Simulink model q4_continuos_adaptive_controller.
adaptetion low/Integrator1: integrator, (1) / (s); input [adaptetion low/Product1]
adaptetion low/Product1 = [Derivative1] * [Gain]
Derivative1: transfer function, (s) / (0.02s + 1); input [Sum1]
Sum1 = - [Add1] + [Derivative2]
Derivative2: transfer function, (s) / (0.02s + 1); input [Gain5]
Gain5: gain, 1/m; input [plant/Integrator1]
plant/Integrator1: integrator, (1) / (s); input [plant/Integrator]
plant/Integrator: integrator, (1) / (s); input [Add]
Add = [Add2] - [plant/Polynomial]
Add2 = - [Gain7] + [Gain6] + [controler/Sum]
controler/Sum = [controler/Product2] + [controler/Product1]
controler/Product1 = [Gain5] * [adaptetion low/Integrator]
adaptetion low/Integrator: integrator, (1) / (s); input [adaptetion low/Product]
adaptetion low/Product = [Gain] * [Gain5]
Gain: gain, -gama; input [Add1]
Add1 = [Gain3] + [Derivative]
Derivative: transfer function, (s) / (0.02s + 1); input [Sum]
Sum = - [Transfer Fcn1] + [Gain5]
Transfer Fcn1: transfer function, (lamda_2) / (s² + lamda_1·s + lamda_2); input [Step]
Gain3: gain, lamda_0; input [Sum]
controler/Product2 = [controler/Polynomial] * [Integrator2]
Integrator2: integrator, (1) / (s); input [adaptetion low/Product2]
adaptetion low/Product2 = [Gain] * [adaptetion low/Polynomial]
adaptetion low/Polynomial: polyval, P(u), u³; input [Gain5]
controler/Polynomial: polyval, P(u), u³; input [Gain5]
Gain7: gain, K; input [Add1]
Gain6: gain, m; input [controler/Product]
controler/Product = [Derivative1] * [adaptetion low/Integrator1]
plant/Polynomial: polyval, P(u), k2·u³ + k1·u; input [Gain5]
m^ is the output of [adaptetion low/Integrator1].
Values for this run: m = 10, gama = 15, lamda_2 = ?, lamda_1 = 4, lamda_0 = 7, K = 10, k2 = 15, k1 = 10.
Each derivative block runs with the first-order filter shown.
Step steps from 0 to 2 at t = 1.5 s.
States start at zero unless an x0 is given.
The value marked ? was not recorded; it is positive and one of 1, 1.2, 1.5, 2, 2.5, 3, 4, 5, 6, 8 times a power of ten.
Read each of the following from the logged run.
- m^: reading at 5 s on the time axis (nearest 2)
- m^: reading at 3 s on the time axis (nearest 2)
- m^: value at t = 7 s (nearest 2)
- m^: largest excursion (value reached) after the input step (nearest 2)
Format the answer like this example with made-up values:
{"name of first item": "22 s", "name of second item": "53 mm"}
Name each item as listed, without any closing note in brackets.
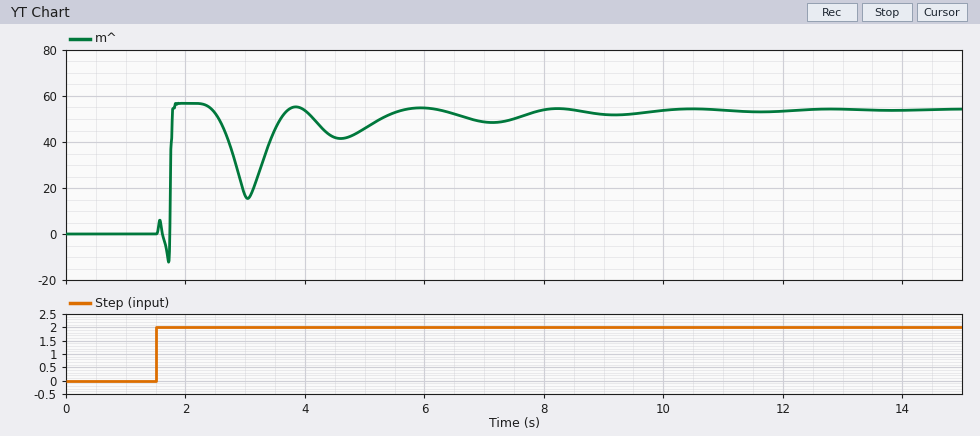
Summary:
{"m^: reading at 5 s on the time axis": "46", "m^: reading at 3 s on the time axis": "16", "m^: value at t = 7 s": "48", "m^: largest excursion (value reached) after the input step": "56"}
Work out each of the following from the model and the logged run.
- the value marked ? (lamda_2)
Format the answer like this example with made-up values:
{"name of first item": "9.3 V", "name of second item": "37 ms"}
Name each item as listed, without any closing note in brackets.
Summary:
{"the value marked ?": "12"}
